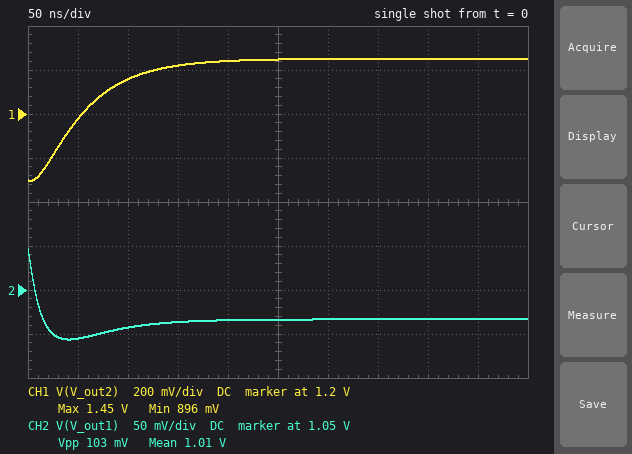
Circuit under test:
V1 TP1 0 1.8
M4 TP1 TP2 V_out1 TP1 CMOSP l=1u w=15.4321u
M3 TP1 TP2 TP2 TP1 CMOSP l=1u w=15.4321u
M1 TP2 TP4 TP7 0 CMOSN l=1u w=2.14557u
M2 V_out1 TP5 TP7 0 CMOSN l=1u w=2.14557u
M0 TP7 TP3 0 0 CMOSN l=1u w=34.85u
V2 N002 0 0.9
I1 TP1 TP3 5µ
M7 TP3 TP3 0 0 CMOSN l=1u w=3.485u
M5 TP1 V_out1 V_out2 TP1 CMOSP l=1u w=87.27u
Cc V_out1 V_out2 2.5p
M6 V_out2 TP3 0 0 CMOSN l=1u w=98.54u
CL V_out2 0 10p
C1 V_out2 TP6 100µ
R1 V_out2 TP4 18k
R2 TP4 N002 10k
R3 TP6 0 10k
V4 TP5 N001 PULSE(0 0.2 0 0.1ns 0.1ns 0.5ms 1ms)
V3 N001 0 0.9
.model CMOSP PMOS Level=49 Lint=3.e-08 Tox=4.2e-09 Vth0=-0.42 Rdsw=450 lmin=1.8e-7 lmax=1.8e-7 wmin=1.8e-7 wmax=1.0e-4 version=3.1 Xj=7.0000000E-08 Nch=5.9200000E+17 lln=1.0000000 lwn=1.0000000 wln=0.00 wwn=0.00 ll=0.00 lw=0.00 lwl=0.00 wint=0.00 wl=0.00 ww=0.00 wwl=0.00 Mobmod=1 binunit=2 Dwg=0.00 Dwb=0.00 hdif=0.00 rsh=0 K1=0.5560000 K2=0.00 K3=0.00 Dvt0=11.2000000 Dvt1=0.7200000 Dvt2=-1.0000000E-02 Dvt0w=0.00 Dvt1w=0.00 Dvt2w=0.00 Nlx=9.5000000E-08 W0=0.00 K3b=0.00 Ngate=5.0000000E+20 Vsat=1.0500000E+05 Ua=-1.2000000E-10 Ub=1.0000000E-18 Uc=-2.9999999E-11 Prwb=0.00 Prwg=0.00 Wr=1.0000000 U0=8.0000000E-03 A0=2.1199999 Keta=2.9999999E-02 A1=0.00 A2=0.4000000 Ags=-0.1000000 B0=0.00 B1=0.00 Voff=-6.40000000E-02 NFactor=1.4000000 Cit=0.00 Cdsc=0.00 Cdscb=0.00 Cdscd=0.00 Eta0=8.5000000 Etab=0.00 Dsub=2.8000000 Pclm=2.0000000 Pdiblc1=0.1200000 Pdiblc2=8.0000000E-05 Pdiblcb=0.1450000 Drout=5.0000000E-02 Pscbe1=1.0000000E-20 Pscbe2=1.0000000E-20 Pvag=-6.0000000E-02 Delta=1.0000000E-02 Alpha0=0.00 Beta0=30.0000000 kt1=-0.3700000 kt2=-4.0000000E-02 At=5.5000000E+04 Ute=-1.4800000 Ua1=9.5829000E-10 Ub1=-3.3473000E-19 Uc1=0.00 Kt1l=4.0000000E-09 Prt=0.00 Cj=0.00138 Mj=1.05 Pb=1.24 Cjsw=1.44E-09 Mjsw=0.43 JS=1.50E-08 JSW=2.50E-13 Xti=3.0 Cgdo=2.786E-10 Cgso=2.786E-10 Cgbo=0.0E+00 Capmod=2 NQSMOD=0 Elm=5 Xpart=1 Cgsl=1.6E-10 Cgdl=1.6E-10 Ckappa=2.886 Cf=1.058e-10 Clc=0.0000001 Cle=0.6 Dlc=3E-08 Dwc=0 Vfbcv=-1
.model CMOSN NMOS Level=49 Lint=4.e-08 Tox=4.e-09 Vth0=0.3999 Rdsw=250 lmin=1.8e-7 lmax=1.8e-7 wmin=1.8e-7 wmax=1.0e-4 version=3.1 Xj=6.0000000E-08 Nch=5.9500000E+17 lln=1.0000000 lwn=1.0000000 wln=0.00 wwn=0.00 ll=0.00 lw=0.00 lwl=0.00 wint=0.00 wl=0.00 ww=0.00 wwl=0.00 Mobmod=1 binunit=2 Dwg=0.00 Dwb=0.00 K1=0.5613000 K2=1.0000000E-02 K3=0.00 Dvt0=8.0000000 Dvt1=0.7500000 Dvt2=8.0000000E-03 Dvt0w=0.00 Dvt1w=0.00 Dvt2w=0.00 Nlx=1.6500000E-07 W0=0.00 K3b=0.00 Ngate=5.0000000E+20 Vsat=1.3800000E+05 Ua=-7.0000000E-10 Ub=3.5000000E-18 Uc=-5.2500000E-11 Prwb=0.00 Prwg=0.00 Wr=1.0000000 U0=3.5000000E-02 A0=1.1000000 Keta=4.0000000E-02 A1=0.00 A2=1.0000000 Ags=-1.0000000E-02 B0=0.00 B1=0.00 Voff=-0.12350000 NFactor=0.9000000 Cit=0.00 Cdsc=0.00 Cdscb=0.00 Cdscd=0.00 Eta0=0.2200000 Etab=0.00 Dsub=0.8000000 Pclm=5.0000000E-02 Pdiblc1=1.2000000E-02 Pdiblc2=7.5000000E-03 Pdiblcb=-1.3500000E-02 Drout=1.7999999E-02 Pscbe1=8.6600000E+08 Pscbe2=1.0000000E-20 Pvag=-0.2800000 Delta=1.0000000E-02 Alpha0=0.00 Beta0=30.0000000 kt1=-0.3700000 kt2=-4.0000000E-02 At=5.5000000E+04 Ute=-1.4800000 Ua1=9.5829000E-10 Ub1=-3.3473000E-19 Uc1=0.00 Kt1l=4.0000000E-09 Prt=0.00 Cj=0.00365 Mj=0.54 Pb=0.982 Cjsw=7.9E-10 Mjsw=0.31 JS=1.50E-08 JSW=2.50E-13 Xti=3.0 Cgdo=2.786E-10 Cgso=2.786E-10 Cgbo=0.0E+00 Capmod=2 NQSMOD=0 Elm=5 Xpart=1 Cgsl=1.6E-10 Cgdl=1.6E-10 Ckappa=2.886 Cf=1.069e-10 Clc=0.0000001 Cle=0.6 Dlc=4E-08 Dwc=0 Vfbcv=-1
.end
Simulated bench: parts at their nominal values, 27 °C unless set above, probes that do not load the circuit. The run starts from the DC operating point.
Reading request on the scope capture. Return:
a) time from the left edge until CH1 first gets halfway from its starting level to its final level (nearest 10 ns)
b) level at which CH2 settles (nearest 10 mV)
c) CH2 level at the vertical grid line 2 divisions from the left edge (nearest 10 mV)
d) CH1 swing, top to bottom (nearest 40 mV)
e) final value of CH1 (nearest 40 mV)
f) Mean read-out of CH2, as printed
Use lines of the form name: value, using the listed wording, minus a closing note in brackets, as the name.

time from the left edge until CH1 first gets halfway from its starting level to its final level: 50 ns
level at which CH2 settles: 1.02 V
CH2 level at the vertical grid line 2 divisions from the left edge: 1.01 V
CH1 swing, top to bottom: 560 mV
final value of CH1: 1.44 V
Mean read-out of CH2, as printed: 1.01 V
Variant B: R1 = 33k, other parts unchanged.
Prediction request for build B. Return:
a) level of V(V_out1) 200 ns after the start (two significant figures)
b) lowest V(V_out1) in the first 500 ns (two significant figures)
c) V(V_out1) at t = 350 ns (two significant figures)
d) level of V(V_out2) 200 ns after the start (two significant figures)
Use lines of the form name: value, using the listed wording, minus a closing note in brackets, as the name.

level of V(V_out1) 200 ns after the start: 950 mV
lowest V(V_out1) in the first 500 ns: 840 mV
V(V_out1) at t = 350 ns: 880 mV
level of V(V_out2) 200 ns after the start: 1.6 V
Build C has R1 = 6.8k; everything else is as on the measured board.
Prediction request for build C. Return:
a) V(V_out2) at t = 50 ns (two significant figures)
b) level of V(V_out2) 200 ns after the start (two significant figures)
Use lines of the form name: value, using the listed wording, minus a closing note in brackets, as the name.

V(V_out2) at t = 50 ns: 1.1 V
level of V(V_out2) 200 ns after the start: 1.2 V
